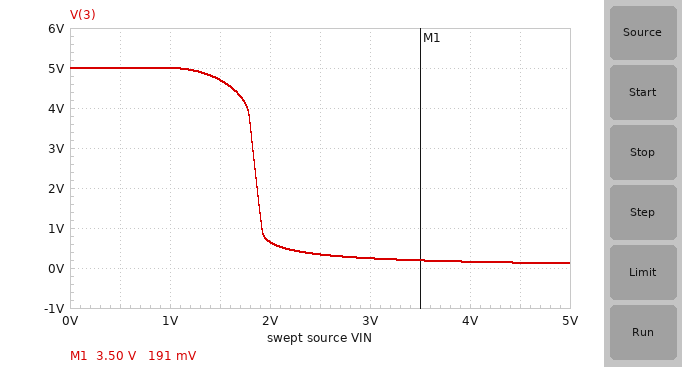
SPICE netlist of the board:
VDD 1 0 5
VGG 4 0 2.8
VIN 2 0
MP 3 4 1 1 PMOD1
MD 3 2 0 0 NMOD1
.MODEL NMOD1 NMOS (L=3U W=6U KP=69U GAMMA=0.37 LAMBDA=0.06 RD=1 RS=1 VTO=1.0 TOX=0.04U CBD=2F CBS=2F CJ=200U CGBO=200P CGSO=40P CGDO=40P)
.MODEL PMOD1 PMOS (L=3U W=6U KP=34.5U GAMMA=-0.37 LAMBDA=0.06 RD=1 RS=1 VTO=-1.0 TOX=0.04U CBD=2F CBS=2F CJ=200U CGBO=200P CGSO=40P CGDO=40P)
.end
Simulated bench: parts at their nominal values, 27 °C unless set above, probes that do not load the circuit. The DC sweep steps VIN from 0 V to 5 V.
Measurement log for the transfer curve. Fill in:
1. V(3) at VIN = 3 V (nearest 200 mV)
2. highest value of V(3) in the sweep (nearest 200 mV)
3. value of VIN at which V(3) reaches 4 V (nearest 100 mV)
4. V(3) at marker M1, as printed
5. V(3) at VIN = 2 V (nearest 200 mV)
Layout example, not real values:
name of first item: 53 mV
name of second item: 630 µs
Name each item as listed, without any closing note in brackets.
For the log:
V(3) at VIN = 3 V: 200 mV
highest value of V(3) in the sweep: 5.0 V
value of VIN at which V(3) reaches 4 V: 1.8 V
V(3) at marker M1, as printed: 191 mV
V(3) at VIN = 2 V: 600 mV
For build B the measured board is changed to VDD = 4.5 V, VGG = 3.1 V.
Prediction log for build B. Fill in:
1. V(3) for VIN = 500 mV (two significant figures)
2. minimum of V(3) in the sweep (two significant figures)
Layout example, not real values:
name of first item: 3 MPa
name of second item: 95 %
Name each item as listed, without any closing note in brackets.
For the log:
V(3) for VIN = 500 mV: 4.5 V
minimum of V(3) in the sweep: 13 mV
